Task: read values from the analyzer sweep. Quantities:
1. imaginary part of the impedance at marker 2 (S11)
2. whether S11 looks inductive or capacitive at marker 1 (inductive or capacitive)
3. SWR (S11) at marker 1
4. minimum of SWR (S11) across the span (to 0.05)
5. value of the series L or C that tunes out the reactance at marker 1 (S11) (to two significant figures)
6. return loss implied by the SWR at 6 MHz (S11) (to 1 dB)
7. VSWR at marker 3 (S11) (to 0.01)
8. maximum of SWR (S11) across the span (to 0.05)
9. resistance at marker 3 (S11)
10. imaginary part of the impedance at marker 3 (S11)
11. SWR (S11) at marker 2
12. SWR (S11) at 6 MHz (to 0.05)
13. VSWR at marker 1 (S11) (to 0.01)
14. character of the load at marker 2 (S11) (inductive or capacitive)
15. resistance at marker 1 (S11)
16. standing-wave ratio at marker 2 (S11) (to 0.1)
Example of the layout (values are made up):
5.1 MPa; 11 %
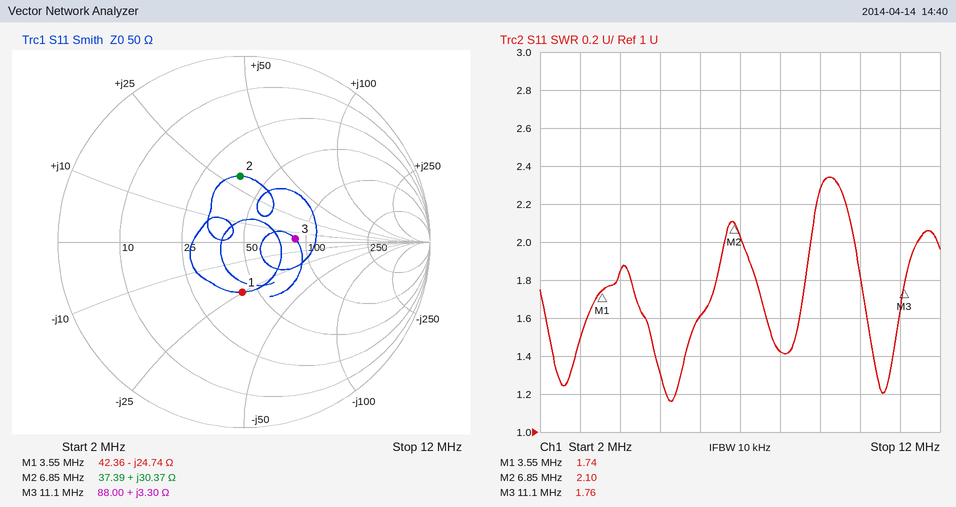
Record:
+30.37 Ω; capacitive; 1.74; 1.15; 1.1 µH; 13 dB; 1.76; 2.35; 88.00 Ω; +3.30 Ω; 2.10; 1.60; 1.74; inductive; 42.36 Ω; 2.1
